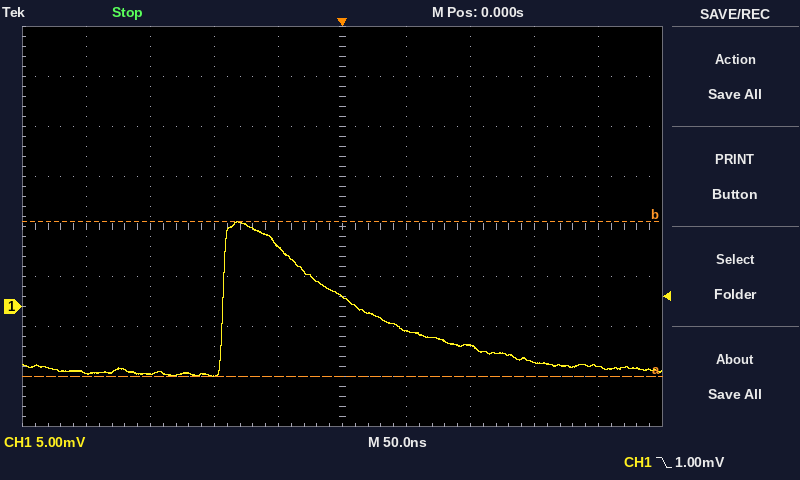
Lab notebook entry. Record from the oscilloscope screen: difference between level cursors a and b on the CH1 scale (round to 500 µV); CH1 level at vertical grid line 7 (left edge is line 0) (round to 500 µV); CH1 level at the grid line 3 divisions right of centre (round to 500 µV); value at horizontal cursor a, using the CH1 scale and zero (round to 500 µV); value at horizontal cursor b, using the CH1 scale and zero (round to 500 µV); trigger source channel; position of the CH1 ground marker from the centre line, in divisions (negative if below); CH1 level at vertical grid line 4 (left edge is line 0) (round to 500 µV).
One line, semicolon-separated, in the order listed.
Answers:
15.5 mV; -4.0 mV; -5.5 mV; -7.0 mV; 8.5 mV; CH1; -1.6 div; 6.0 mV
